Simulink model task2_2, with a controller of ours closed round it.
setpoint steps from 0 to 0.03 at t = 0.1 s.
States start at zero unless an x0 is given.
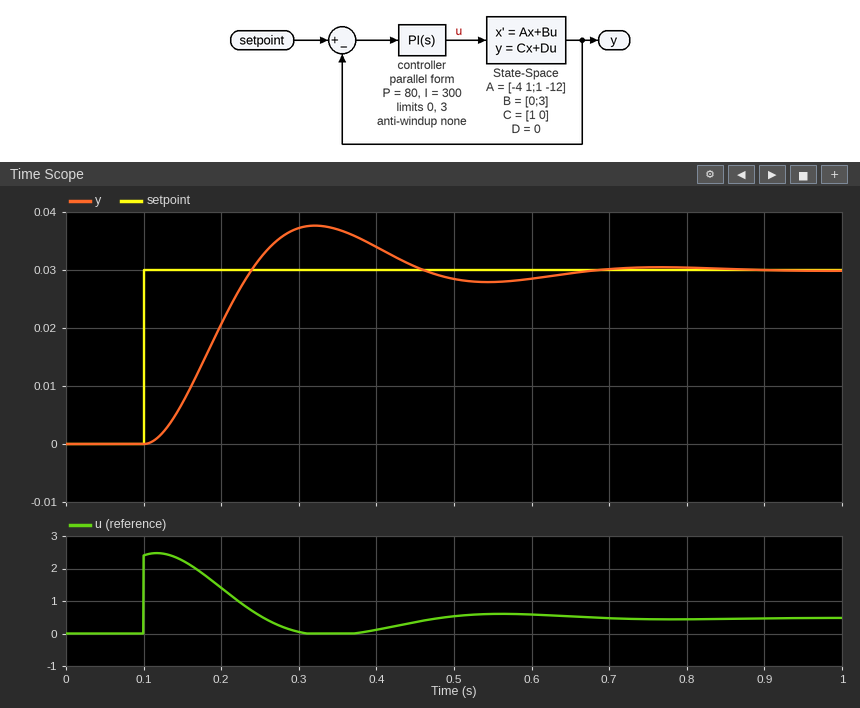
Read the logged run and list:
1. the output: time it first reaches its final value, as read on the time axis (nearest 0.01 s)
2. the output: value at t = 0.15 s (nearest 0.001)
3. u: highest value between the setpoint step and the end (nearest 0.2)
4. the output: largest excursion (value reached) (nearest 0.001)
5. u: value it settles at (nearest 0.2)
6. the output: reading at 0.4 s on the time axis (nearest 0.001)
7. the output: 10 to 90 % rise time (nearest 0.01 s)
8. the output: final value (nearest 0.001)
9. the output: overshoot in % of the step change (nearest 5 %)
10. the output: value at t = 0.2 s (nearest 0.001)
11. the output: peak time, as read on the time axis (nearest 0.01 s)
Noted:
0.24 s
0.007
2.4
0.038
0.4
0.034
0.09 s
0.030
25 %
0.021
0.32 s
